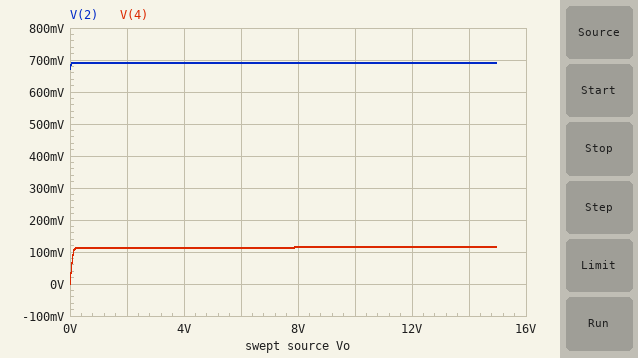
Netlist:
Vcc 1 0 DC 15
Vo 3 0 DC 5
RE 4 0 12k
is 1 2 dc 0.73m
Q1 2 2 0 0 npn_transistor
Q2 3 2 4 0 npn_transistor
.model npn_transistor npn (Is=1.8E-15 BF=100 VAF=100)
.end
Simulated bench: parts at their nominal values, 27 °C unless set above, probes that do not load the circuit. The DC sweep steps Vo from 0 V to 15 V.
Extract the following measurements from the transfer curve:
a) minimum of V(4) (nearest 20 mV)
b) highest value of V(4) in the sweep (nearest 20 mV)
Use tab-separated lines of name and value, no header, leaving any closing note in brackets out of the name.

minimum of V(4)	0 V
highest value of V(4) in the sweep	120 mV
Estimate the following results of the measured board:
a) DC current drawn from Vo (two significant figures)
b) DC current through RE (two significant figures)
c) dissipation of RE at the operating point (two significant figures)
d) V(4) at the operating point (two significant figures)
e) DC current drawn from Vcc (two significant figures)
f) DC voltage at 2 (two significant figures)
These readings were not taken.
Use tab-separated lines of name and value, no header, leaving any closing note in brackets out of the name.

DC current drawn from Vo	9.4 µA
DC current through RE	9.5 µA
dissipation of RE at the operating point	1.1 µW
V(4) at the operating point	110 mV
DC current drawn from Vcc	730 µA
DC voltage at 2	690 mV
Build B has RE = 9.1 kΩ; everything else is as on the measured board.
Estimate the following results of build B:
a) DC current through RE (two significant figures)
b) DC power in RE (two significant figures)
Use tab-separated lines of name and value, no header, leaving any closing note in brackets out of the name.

DC current through RE	12 µA
DC power in RE	1.3 µW
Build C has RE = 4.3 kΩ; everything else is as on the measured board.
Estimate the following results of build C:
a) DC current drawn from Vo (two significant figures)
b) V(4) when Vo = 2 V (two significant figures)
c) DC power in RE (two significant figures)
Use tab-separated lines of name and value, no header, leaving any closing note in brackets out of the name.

DC current drawn from Vo	21 µA
V(4) when Vo = 2 V	92 mV
DC power in RE	2.0 µW
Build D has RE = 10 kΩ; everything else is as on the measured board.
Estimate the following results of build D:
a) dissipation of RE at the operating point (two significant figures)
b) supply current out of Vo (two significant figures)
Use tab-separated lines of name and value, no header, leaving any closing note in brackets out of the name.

dissipation of RE at the operating point	1.2 µW
supply current out of Vo	11 µA
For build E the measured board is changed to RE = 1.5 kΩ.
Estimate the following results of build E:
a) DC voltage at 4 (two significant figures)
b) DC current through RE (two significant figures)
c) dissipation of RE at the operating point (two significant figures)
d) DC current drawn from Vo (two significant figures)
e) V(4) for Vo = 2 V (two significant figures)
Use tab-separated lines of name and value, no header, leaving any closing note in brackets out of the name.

DC voltage at 4	72 mV
DC current through RE	48 µA
dissipation of RE at the operating point	3.4 µW
DC current drawn from Vo	47 µA
V(4) for Vo = 2 V	71 mV
